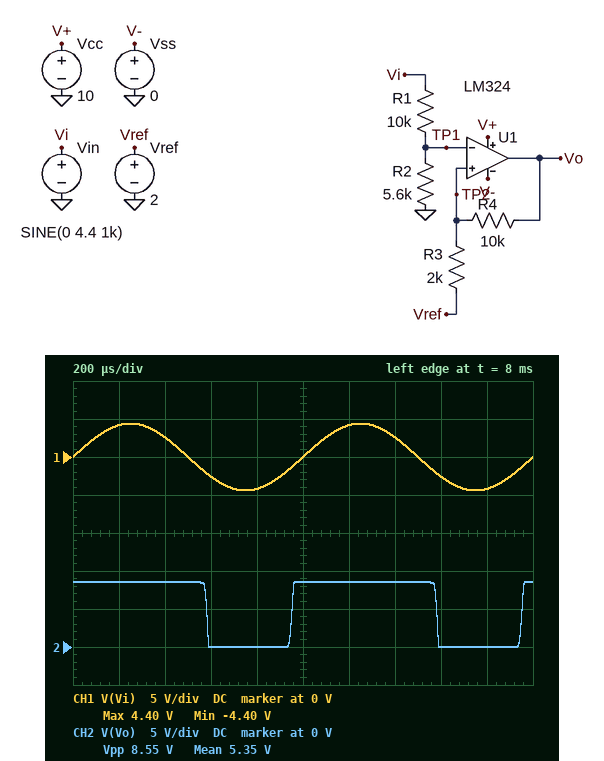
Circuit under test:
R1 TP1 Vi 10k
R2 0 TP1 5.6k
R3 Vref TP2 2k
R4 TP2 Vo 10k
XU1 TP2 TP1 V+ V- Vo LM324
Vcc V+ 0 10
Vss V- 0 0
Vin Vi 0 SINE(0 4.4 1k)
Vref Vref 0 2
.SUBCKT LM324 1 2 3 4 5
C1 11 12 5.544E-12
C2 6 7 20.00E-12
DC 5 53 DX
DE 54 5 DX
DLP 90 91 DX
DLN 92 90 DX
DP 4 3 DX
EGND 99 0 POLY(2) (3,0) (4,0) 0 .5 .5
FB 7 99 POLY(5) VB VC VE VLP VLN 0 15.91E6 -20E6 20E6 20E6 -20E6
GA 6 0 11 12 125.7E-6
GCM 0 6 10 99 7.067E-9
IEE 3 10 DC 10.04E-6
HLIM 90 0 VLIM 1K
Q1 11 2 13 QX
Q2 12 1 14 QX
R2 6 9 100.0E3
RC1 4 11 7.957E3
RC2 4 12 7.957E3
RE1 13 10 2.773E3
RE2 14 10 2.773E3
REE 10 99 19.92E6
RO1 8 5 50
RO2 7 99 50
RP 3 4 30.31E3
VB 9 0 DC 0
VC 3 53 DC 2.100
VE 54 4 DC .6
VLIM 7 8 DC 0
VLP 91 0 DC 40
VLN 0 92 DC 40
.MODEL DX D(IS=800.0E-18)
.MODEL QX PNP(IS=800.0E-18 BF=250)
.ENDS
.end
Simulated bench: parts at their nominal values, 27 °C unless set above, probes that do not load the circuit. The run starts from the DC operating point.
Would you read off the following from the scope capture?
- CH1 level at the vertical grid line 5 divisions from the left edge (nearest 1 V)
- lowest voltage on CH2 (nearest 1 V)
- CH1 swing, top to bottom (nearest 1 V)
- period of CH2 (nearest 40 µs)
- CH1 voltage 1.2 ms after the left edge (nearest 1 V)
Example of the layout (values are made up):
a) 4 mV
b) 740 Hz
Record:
a) 0 V
b) 0 V
c) 9 V
d) 1.00 ms
e) 4 V
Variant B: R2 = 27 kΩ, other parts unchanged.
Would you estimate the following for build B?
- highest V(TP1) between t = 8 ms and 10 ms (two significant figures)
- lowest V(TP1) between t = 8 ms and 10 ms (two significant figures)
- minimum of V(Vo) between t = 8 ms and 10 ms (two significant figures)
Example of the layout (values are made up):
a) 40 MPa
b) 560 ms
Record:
a) 3.2 V
b) -2.0 V
c) -67 mV
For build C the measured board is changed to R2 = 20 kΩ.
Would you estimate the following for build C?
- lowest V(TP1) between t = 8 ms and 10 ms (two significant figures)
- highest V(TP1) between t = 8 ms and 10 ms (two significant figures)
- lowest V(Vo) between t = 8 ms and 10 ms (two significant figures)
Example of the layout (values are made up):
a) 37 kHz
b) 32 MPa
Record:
a) -1.9 V
b) 2.9 V
c) -65 mV
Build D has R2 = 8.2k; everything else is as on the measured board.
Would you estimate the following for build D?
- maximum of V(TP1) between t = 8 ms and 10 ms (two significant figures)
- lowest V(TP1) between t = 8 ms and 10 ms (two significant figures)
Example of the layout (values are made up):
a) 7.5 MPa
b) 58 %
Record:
a) 2.0 V
b) -1.5 V
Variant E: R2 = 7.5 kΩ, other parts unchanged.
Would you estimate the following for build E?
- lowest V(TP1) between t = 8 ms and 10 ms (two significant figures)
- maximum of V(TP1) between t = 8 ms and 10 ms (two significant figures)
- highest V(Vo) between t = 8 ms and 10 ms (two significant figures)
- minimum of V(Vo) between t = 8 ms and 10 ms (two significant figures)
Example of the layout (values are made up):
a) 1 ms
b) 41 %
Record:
a) -1.4 V
b) 1.9 V
c) 8.5 V
d) -54 mV
